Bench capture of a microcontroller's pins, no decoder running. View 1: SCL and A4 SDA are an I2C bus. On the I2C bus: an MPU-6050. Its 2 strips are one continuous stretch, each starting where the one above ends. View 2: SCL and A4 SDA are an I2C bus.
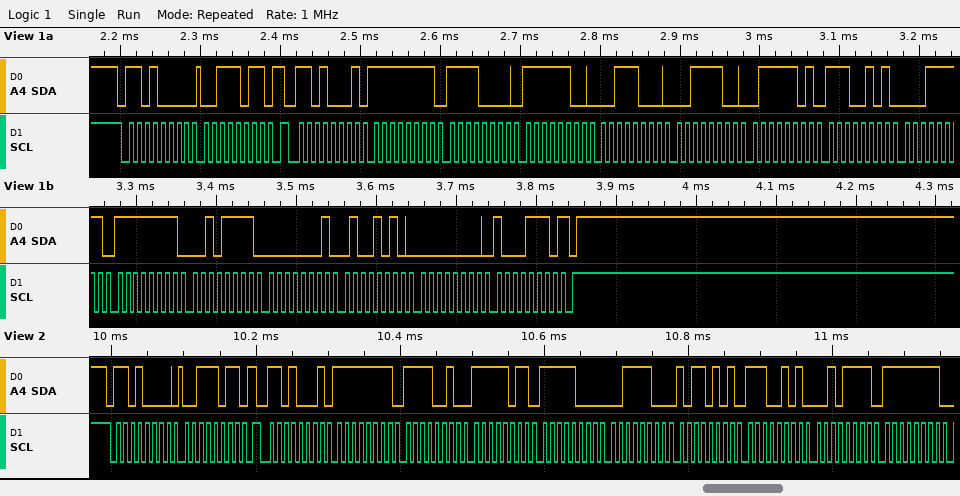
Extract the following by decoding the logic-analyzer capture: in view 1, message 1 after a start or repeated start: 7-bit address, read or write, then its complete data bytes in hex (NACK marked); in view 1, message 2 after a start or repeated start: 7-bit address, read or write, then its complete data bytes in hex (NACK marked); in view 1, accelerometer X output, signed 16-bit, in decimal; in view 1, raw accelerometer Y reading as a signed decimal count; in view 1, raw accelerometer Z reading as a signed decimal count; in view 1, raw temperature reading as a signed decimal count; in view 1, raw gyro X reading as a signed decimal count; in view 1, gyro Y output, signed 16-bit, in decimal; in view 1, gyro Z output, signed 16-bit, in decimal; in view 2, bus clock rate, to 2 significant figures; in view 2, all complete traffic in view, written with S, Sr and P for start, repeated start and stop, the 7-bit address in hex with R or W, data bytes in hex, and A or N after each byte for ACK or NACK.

0x68 write: 3B
0x68 read: FF F0 FC 38 3C 7D E5 1F FF 2F 01 4A 00 8E NACK
-16
-968
15485
-6881
-209
330
142
100 kHz
S 68W A 3B A Sr 68R A FF A F2 A FB A F8 A 3C A B5 A E5 A 2F A FF A
